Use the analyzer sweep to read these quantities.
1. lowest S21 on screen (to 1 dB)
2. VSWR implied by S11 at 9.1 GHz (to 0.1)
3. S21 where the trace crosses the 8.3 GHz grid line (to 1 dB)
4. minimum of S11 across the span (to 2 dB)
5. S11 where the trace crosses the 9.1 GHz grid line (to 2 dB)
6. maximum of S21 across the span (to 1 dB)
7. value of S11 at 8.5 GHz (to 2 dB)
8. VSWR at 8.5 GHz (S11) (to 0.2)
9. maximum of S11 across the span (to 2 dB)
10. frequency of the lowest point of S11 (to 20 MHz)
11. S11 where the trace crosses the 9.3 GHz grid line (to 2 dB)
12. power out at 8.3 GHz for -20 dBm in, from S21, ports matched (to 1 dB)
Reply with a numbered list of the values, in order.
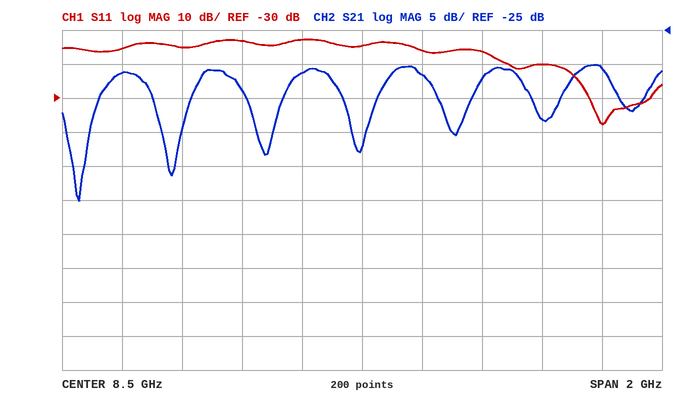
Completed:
1. -50 dB
2. 1.2
3. -31 dB
4. -38 dB
5. -20 dB
6. -30 dB
7. -14 dB
8. 1.4
9. -12 dB
10. 9.30 GHz
11. -38 dB
12. -51 dBm
